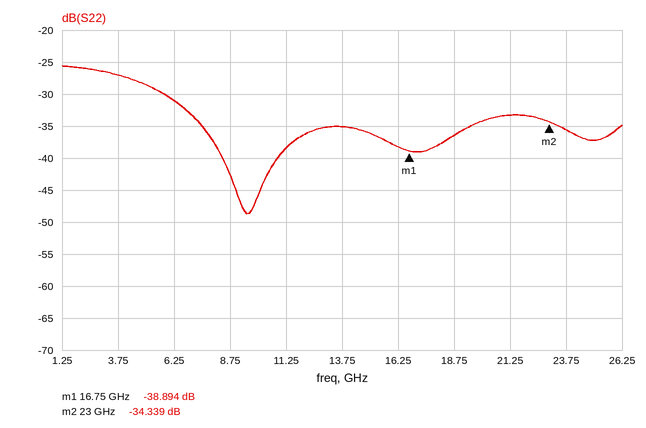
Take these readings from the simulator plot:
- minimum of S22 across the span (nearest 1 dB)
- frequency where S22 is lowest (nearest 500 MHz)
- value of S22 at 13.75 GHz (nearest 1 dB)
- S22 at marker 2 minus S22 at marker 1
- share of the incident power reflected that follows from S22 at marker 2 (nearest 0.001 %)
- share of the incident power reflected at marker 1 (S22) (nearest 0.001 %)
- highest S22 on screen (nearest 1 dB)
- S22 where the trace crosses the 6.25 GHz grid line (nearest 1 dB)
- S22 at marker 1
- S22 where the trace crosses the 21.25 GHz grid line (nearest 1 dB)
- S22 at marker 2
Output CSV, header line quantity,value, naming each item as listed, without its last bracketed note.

quantity,value
minimum of S22 across the span,-49 dB
frequency where S22 is lowest,9.5 GHz
value of S22 at 13.75 GHz,-35 dB
S22 at marker 2 minus S22 at marker 1,4.555 dB
share of the incident power reflected that follows from S22 at marker 2,0.037 %
share of the incident power reflected at marker 1 (S22),0.013 %
highest S22 on screen,-26 dB
S22 where the trace crosses the 6.25 GHz grid line,-31 dB
S22 at marker 1,-38.894 dB
S22 where the trace crosses the 21.25 GHz grid line,-33 dB
S22 at marker 2,-34.339 dB
